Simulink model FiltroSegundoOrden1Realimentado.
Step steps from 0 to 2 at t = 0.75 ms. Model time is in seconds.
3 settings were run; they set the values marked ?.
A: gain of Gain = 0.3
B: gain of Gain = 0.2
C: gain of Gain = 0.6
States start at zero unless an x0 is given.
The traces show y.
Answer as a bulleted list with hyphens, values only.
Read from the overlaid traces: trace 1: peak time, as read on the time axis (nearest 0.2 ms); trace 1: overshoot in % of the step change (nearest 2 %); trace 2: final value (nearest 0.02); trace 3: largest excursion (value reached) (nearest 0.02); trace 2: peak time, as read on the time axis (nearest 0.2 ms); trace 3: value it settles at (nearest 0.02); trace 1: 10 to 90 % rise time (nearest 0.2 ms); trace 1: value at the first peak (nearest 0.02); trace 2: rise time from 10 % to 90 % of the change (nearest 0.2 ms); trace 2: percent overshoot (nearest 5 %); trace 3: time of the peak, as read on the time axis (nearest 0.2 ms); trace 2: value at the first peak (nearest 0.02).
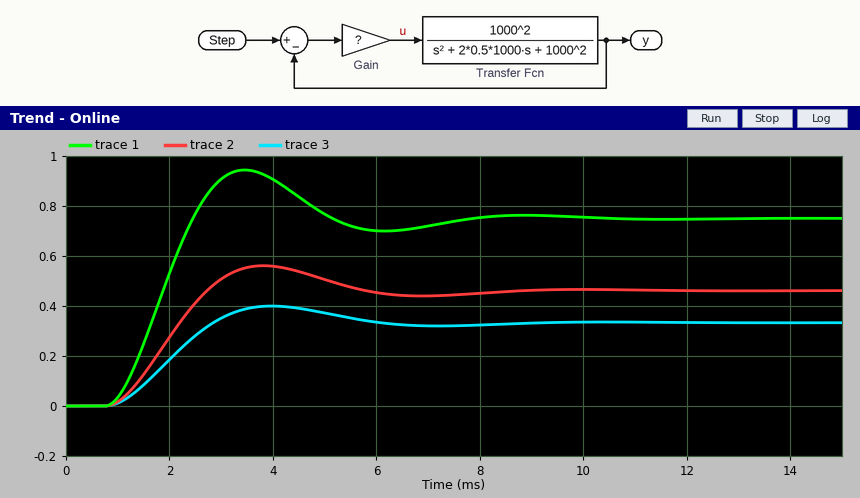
- 3.4 ms
- 26 %
- 0.46
- 0.40
- 3.8 ms
- 0.34
- 1.2 ms
- 0.94
- 1.4 ms
- 20 %
- 4.0 ms
- 0.56
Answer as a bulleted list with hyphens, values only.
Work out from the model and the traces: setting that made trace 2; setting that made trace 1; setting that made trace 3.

- A
- C
- B
